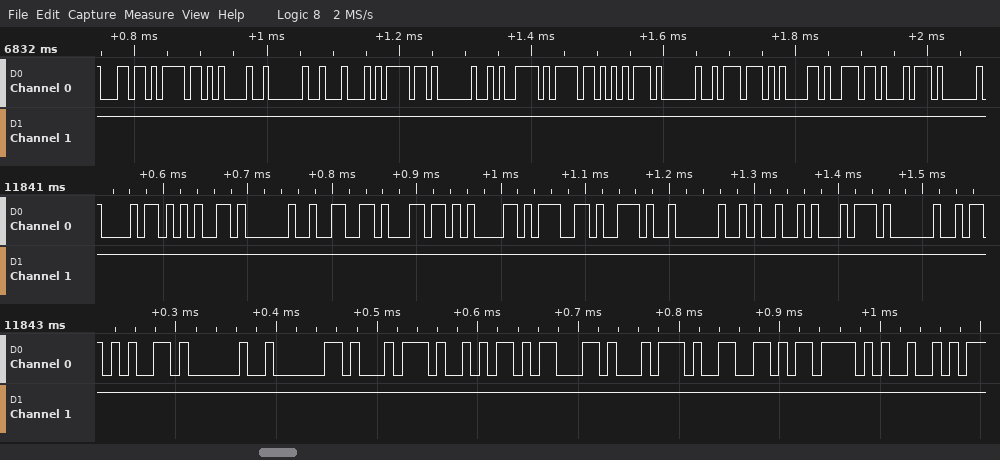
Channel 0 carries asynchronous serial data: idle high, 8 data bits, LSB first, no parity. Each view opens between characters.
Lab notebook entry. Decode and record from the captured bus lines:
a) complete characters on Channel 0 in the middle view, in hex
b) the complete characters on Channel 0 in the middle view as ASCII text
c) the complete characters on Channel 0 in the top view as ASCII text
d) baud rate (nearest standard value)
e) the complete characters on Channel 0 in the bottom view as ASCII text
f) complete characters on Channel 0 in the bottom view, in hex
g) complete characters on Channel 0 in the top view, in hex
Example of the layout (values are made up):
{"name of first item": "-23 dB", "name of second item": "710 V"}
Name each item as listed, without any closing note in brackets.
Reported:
{"complete characters on Channel 0 in the middle view, in hex": "68, 65, 20, 66, 6C, 61, 67, 2E, 20, 49, 74, 20", "the complete characters on Channel 0 in the middle view as ASCII text": "\"he flag. It \"", "the complete characters on Channel 0 in the top view as ASCII text": "\"lo! Do you want\"", "baud rate": "115200 baud", "the complete characters on Channel 0 in the bottom view as ASCII text": "\"e `tjctf{I\"", "complete characters on Channel 0 in the bottom view, in hex": "65, 20, 60, 74, 6A, 63, 74, 66, 7B, 49", "complete characters on Channel 0 in the top view, in hex": "6C, 6F, 21, 20, 44, 6F, 20, 79, 6F, 75, 20, 77, 61, 6E, 74"}
